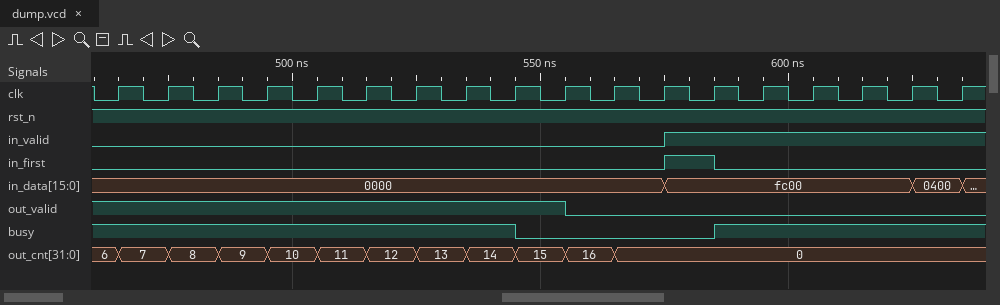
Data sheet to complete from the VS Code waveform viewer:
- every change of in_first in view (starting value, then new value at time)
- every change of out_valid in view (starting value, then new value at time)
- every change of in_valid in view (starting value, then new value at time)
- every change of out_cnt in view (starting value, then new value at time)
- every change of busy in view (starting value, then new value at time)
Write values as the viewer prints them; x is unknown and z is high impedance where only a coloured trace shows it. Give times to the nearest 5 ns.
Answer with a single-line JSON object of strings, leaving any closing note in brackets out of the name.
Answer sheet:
{"every change of in_first in view": "0, 1 at 575 ns, 0 at 585 ns", "every change of out_valid in view": "1, 0 at 555 ns", "every change of in_valid in view": "0, 1 at 575 ns", "every change of out_cnt in view": "6, 7 at 465 ns, 8 at 475 ns, 9 at 485 ns, 10 at 495 ns, 11 at 505 ns, 12 at 515 ns, 13 at 525 ns, 14 at 535 ns, 15 at 545 ns, 16 at 555 ns, 0 at 565 ns", "every change of busy in view": "1, 0 at 545 ns, 1 at 585 ns"}
